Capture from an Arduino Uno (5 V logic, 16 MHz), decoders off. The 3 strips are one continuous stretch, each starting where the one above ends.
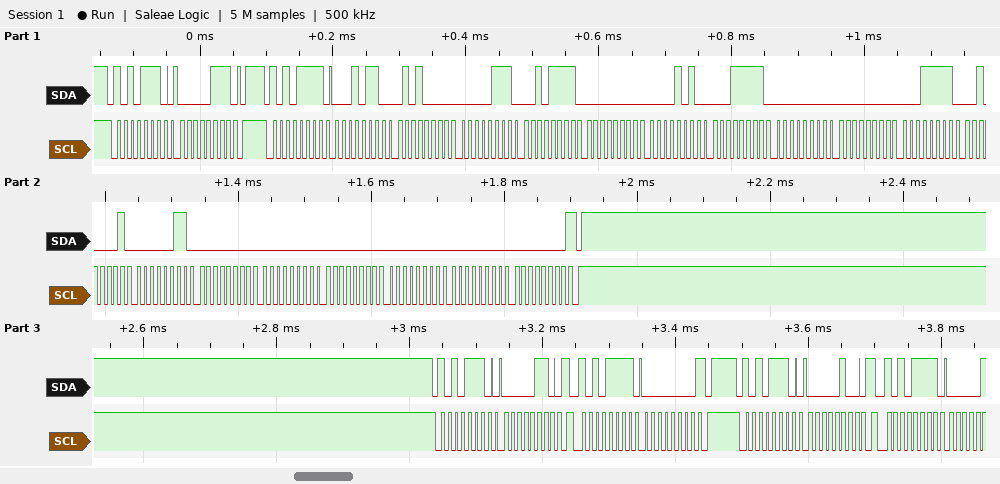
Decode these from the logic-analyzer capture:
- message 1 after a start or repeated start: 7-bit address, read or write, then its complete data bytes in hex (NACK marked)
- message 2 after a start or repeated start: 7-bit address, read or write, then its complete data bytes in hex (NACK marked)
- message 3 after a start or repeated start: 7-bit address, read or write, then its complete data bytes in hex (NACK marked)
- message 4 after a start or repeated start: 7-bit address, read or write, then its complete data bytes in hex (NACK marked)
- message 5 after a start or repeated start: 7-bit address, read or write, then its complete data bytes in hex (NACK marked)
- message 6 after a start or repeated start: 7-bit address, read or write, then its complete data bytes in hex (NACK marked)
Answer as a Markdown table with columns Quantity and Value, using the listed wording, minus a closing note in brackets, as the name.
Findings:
| Quantity | Value |
|---|---|
| message 1 after a start or repeated start: 7-bit address, read or write, then its complete data bytes in hex | 0x57 write: 07 |
| message 2 after a start or repeated start: 7-bit address, read or write, then its complete data bytes in hex | 0x57 read: 16 50 07 2F 00 0A 1F 00 00 1F 21 03 00 00 00 00 00 00 NACK |
| message 3 after a start or repeated start: 7-bit address, read or write, then its complete data bytes in hex | 0x57 write: 06 |
| message 4 after a start or repeated start: 7-bit address, read or write, then its complete data bytes in hex | 0x57 read: 00 NACK |
| message 5 after a start or repeated start: 7-bit address, read or write, then its complete data bytes in hex | 0x57 write: 04 |
| message 6 after a start or repeated start: 7-bit address, read or write, then its complete data bytes in hex | 0x57 read |
